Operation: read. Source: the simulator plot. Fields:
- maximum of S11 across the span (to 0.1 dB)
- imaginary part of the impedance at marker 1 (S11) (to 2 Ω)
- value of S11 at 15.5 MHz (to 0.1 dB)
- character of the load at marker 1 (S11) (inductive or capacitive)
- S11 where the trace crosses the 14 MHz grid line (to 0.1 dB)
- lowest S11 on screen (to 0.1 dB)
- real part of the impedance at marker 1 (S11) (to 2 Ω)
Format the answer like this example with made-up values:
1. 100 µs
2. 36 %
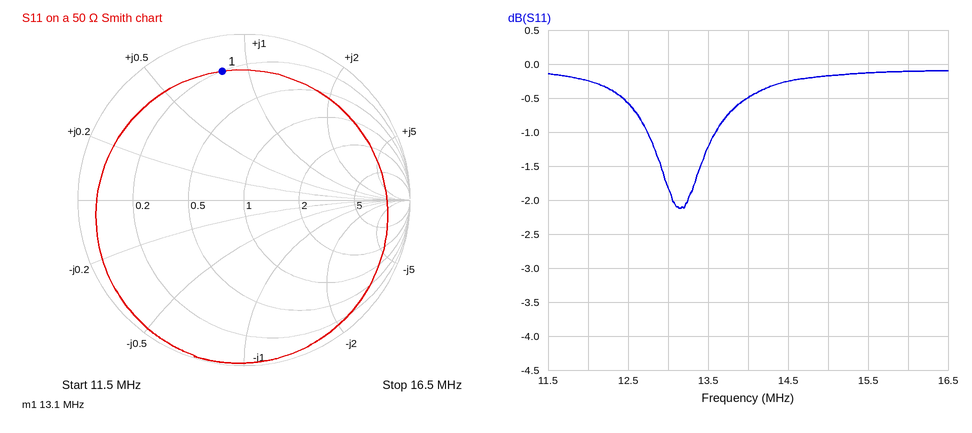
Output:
1. -0.1 dB
2. +42 Ω
3. -0.1 dB
4. inductive
5. -0.5 dB
6. -2.1 dB
7. 10 Ω
